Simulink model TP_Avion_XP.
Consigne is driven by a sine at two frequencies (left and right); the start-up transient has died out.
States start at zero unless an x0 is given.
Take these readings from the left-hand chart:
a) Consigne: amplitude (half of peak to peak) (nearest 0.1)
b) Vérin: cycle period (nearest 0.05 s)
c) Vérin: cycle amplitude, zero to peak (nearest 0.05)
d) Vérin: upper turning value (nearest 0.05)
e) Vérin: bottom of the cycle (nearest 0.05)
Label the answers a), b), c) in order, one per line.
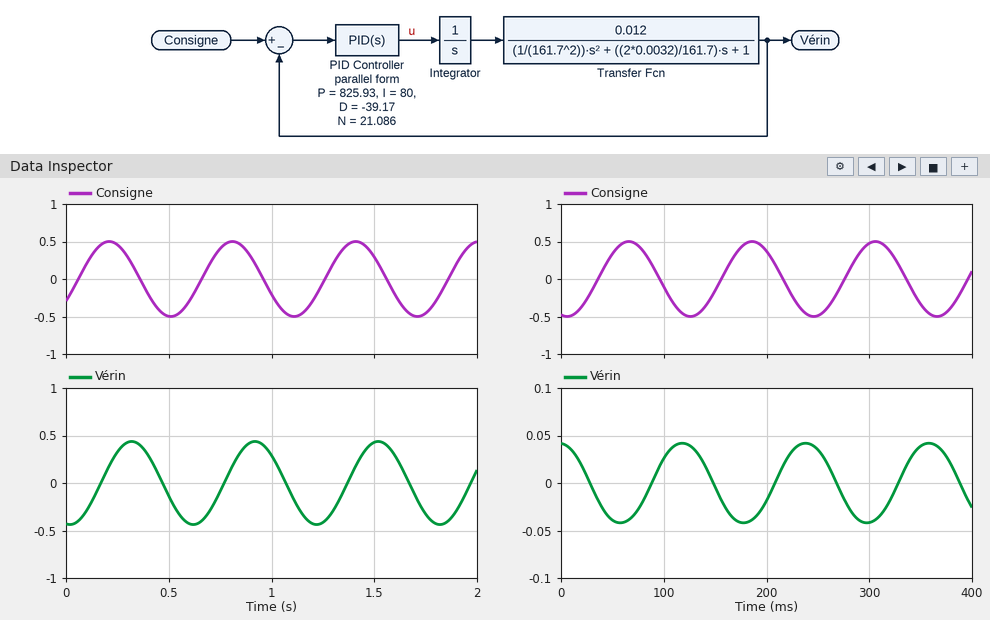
a) 0.5
b) 0.60 s
c) 0.45
d) 0.45
e) -0.45
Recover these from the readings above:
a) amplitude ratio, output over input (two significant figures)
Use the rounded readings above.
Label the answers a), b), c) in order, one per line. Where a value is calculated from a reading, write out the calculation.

a) 0.45 / 0.5 = 0.90
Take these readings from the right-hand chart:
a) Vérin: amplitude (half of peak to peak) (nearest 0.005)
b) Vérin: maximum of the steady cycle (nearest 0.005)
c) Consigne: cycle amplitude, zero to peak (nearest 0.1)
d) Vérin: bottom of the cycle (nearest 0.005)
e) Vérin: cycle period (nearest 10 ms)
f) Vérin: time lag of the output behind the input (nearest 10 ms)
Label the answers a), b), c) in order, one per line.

a) 0.040
b) 0.040
c) 0.5
d) -0.040
e) 120 ms
f) 50 ms
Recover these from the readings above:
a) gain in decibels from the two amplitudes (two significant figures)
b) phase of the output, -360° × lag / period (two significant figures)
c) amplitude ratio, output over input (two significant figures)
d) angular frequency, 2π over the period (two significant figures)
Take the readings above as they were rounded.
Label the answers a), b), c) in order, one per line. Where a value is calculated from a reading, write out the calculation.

a) 20 log10(0.04 / 0.5) = -22 dB
b) -360 × 50 / 120 = -150°
c) 0.04 / 0.5 = 0.080
d) 2π / 120 = 0.052 rad/ms
